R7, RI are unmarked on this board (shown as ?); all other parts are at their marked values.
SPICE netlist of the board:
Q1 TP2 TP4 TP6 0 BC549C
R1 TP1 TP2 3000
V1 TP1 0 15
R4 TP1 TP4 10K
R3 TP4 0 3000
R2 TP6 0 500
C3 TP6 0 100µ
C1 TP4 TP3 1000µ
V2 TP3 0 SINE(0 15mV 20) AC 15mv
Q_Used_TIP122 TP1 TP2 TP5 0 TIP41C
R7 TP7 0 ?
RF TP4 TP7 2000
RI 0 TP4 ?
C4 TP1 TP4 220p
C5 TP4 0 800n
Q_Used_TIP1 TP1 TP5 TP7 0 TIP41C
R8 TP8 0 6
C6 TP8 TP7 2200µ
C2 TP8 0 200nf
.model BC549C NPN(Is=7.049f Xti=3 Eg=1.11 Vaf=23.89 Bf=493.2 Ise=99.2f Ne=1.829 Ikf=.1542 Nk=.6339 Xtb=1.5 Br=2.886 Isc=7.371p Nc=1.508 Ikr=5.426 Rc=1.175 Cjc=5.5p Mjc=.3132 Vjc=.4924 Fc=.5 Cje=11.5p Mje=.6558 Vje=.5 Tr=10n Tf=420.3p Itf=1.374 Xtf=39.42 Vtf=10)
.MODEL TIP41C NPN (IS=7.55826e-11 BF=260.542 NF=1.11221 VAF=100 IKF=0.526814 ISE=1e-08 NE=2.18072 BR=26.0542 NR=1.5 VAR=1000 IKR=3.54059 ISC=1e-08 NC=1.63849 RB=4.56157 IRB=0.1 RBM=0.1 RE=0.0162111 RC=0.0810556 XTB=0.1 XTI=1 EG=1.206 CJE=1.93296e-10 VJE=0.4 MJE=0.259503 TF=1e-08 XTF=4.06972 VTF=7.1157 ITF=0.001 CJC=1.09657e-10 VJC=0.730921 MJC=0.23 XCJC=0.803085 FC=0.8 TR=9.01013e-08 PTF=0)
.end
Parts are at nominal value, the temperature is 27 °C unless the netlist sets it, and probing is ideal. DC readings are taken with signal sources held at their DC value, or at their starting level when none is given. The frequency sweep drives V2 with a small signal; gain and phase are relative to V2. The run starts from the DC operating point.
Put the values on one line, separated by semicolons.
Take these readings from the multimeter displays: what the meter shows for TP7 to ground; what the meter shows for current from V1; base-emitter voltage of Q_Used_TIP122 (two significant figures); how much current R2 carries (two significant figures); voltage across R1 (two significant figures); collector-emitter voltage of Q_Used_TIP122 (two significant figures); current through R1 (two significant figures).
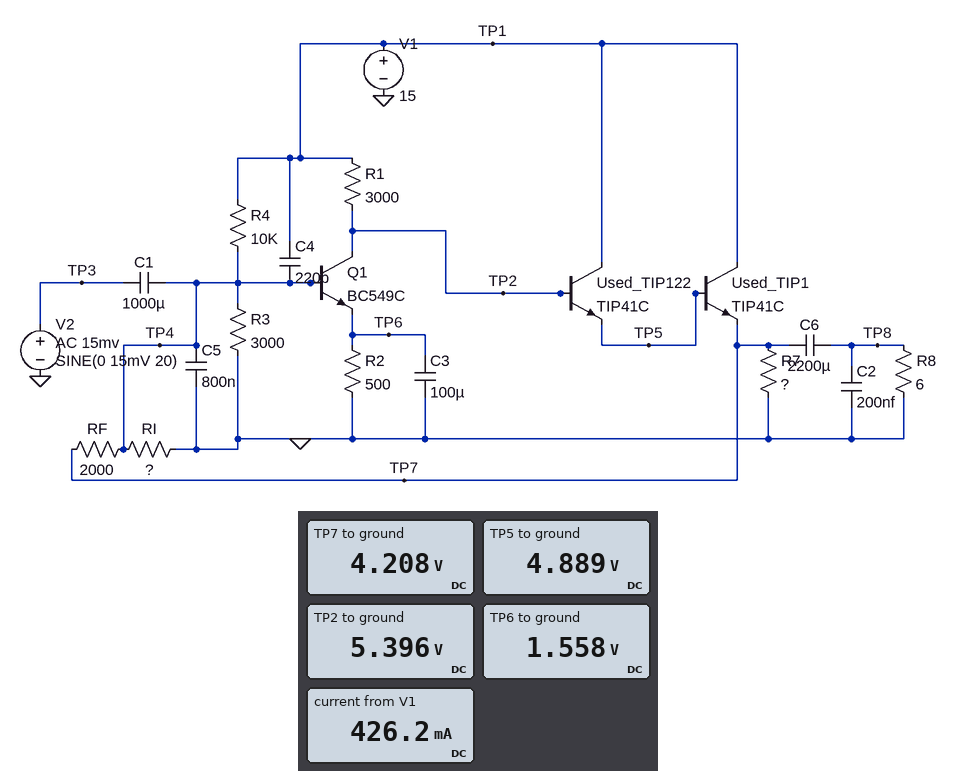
4.208 V; 426.2 mA; 510 mV; 3.1 mA; 9.6 V; 10 V; 3.2 mA
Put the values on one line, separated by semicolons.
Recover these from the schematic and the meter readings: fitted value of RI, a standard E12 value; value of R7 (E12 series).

1.5 kΩ; 10 Ω
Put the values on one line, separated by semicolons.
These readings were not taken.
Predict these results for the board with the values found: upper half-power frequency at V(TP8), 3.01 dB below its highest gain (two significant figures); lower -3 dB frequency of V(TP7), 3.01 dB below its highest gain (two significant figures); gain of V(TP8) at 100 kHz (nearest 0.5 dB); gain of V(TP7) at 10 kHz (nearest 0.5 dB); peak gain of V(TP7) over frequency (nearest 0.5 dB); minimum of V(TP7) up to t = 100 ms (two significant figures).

230 kHz; 160 kHz; 49.0 dB; 47.0 dB; 55.5 dB; 3.8 V
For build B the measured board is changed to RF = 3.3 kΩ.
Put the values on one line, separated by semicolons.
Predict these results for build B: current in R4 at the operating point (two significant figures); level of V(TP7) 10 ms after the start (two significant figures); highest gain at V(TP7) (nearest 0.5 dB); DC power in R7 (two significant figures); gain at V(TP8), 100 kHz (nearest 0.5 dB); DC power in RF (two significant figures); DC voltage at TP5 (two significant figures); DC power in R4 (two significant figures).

1.3 mA; 4.6 V; 54.5 dB; 2.4 W; 48.5 dB; 2.3 mW; 5.6 V; 17 mW
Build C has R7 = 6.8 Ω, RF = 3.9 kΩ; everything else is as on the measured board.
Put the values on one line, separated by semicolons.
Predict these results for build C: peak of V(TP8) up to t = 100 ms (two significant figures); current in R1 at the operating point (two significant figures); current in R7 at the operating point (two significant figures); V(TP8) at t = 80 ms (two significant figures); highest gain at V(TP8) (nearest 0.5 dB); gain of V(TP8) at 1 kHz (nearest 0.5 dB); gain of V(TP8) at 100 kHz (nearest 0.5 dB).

370 mV; 2.9 mA; 750 mA; 250 mV; 52.0 dB; 46.0 dB; 48.0 dB
